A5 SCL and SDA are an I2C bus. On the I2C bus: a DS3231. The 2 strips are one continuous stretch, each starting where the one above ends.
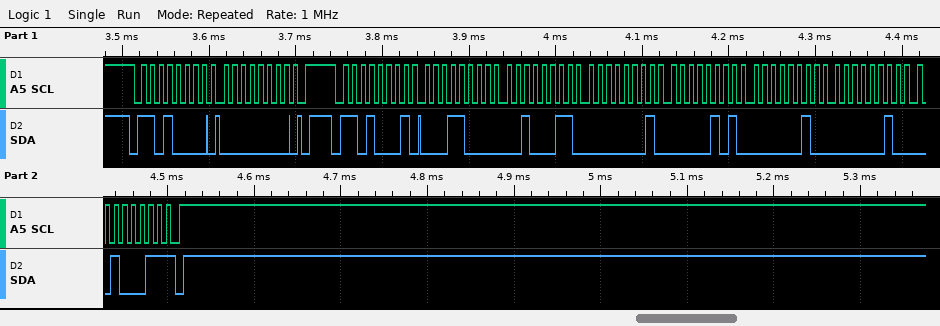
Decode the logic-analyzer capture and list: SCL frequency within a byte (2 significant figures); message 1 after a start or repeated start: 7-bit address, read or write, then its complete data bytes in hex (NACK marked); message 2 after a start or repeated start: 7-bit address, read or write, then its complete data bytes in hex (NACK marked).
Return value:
100 kHz
0x68 write: 00
0x68 read: 18 23 01 05 02 02 23 NACK
